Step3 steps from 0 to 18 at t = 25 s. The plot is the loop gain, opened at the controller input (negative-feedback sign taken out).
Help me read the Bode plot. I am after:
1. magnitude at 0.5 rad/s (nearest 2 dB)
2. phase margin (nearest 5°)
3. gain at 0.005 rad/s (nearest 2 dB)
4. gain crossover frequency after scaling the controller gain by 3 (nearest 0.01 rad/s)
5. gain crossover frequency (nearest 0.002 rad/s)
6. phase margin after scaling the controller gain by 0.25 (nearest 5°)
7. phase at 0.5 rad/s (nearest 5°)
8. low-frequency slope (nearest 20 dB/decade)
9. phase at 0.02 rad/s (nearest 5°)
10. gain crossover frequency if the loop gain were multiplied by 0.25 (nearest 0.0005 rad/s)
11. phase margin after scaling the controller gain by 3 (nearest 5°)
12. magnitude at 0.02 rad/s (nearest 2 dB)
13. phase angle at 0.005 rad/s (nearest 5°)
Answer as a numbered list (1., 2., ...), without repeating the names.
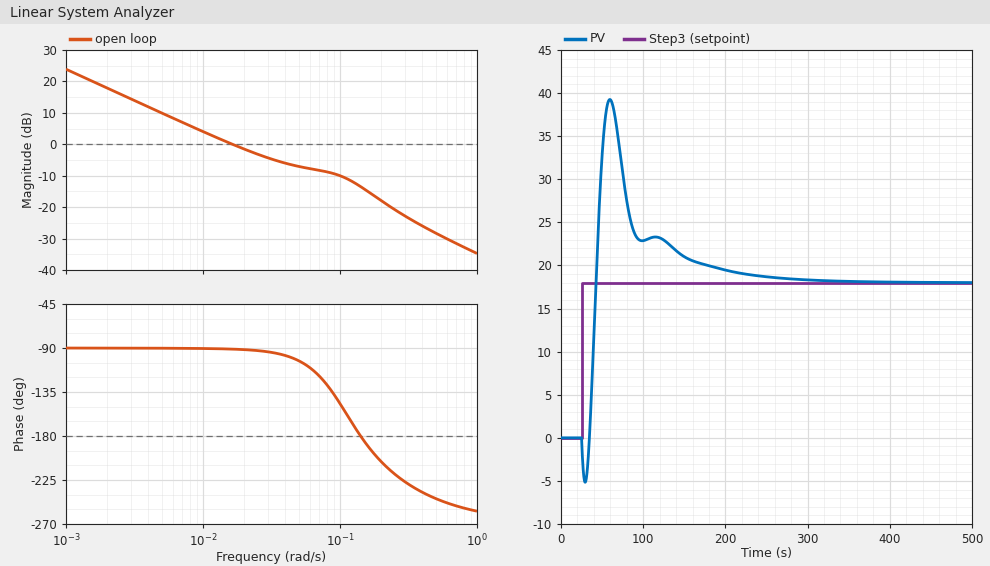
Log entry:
1. -28 dB
2. 90°
3. 10 dB
4. 0.09 rad/s
5. 0.016 rad/s
6. 90°
7. -245°
8. -20 dB/decade
9. -90°
10. 0.0040 rad/s
11. 40°
12. -2 dB
13. -90°
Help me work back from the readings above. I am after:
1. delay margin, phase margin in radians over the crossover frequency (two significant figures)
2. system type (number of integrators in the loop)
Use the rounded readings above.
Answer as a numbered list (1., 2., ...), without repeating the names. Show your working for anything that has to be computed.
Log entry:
1. 90 × π / 180 / 0.016 = 98 s
2. 1
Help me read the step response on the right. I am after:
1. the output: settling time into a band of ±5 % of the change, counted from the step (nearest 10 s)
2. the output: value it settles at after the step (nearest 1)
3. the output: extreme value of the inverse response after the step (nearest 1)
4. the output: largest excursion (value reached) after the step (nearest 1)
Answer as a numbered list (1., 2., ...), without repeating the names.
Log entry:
1. 210 s
2. 18
3. -5
4. 39
